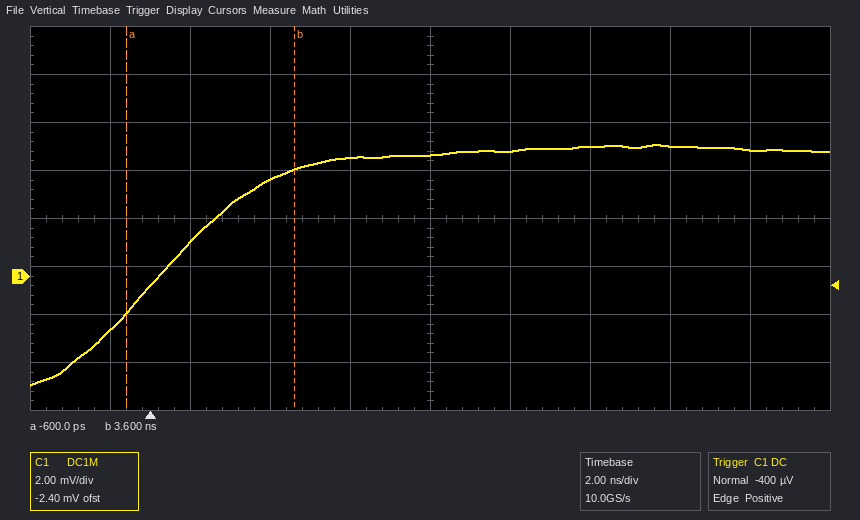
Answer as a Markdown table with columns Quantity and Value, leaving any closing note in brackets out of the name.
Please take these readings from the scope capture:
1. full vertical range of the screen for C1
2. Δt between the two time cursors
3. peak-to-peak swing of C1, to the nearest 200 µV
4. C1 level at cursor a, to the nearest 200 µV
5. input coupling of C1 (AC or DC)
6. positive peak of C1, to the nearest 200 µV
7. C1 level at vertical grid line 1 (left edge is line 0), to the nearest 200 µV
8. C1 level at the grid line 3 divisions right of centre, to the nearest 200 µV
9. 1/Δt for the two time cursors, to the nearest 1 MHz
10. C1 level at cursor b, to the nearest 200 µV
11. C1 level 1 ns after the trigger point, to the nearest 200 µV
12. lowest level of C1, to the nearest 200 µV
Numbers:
| Quantity | Value |
|---|---|
| full vertical range of the screen for C1 | 16 mV |
| Δt between the two time cursors | 4.2 ns |
| peak-to-peak swing of C1, to the nearest 200 µV | 10.0 mV |
| C1 level at cursor a, to the nearest 200 µV | -1.6 mV |
| input coupling of C1 | DC |
| positive peak of C1, to the nearest 200 µV | 5.4 mV |
| C1 level at vertical grid line 1 (left edge is line 0), to the nearest 200 µV | -2.2 mV |
| C1 level at the grid line 3 divisions right of centre, to the nearest 200 µV | 5.4 mV |
| 1/Δt for the two time cursors, to the nearest 1 MHz | 238 MHz |
| C1 level at cursor b, to the nearest 200 µV | 4.4 mV |
| C1 level 1 ns after the trigger point, to the nearest 200 µV | 1.4 mV |
| lowest level of C1, to the nearest 200 µV | -4.6 mV |
